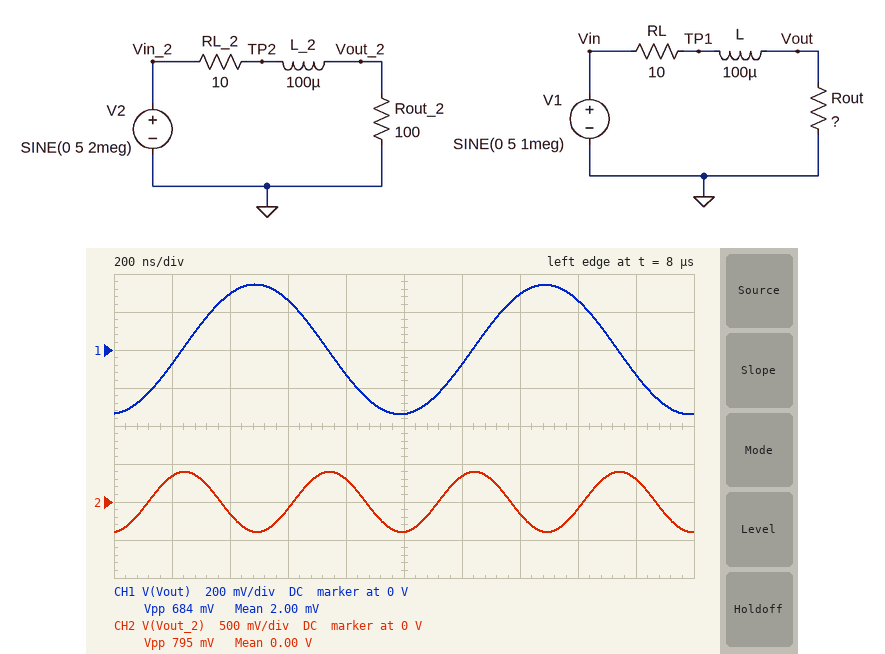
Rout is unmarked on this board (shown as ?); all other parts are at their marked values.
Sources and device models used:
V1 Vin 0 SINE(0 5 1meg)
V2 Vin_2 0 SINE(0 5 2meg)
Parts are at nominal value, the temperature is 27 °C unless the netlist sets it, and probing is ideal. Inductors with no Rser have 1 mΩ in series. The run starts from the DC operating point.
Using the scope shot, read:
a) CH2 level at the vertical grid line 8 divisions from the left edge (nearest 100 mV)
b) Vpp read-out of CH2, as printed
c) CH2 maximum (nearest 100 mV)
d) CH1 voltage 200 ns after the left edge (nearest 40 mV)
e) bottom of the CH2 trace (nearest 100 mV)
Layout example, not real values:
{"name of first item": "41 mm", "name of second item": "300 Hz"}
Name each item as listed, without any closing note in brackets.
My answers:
{"CH2 level at the vertical grid line 8 divisions from the left edge": "-100 mV", "Vpp read-out of CH2, as printed": "795 mV", "CH2 maximum": "400 mV", "CH1 voltage 200 ns after the left edge": "-80 mV", "bottom of the CH2 trace": "-400 mV"}
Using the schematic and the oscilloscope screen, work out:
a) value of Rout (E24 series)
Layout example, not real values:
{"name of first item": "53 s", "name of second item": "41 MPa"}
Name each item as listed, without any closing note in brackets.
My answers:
{"value of Rout": "43 Ω"}
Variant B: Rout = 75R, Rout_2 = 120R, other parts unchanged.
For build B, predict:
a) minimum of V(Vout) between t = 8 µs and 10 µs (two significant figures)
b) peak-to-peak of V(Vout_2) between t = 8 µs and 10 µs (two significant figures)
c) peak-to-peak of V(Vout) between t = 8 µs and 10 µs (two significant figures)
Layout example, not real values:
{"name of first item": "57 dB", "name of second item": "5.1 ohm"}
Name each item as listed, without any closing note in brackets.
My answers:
{"minimum of V(Vout) between t = 8 µs and 10 µs": "-590 mV", "peak-to-peak of V(Vout_2) between t = 8 µs and 10 µs": "950 mV", "peak-to-peak of V(Vout) between t = 8 µs and 10 µs": "1.2 V"}
